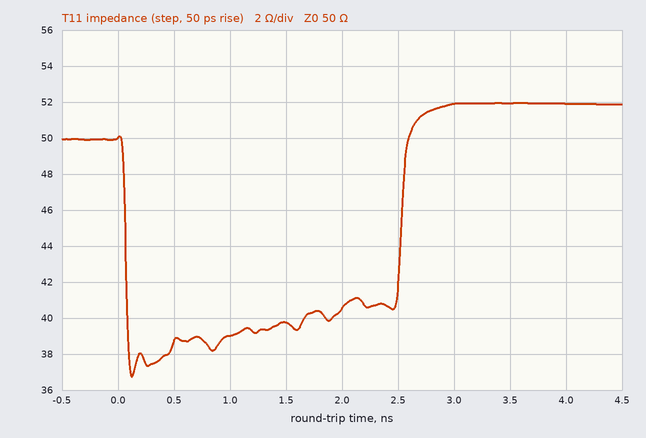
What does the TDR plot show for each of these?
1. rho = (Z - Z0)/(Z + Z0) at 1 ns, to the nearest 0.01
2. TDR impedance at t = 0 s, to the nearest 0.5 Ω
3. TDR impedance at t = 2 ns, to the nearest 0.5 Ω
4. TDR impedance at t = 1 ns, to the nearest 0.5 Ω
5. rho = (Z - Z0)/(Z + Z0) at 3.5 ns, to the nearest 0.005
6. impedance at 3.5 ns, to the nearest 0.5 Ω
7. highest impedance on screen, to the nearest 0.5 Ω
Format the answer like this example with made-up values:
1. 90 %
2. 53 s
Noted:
1. -0.12
2. 50.0 Ω
3. 40.5 Ω
4. 39.0 Ω
5. +0.020
6. 52.0 Ω
7. 52.0 Ω
